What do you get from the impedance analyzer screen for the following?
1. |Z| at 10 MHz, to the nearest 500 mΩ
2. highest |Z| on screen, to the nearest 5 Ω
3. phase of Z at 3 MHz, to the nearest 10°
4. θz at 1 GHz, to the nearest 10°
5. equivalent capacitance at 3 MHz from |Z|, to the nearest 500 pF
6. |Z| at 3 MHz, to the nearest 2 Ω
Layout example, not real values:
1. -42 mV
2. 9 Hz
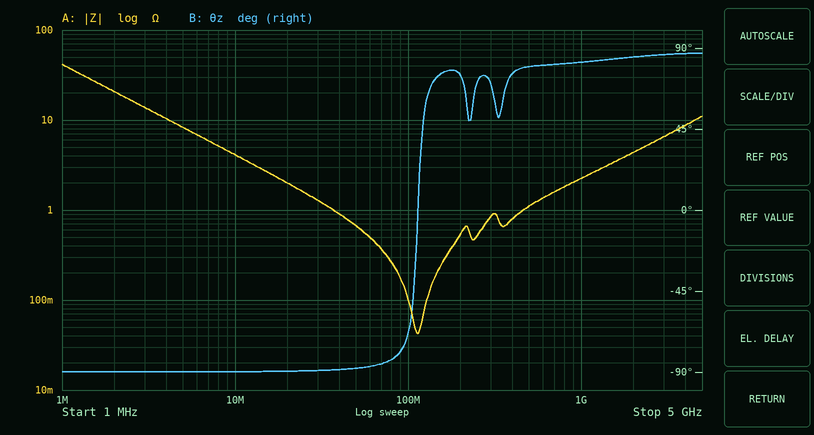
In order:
1. 4.0 Ω
2. 40 Ω
3. -90°
4. 80°
5. 4.0 nF
6. 14 Ω
